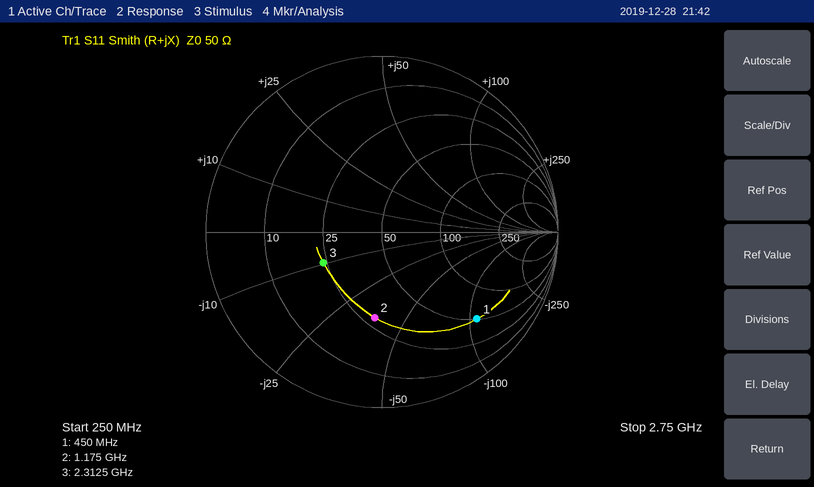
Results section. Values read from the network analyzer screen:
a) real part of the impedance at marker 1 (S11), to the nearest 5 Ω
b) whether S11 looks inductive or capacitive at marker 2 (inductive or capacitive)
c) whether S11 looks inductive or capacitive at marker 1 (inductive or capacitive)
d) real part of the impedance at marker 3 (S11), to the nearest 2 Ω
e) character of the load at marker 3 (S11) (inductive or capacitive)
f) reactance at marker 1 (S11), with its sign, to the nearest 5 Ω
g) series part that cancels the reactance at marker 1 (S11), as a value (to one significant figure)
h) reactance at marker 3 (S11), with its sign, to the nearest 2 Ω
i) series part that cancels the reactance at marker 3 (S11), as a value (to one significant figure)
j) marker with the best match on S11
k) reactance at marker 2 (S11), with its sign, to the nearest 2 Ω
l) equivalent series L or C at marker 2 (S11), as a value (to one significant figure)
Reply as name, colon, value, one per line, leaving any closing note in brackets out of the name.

real part of the impedance at marker 1 (S11), to the nearest 5 Ω: 50 Ω
whether S11 looks inductive or capacitive at marker 2: capacitive
whether S11 looks inductive or capacitive at marker 1: capacitive
real part of the impedance at marker 3 (S11), to the nearest 2 Ω: 24 Ω
character of the load at marker 3 (S11): capacitive
reactance at marker 1 (S11), with its sign, to the nearest 5 Ω: -110 Ω
series part that cancels the reactance at marker 1 (S11), as a value: 40 nH
reactance at marker 3 (S11), with its sign, to the nearest 2 Ω: -10 Ω
series part that cancels the reactance at marker 3 (S11), as a value: 700 pH
marker with the best match on S11: marker 3
reactance at marker 2 (S11), with its sign, to the nearest 2 Ω: -36 Ω
equivalent series L or C at marker 2 (S11), as a value: 4 pF
